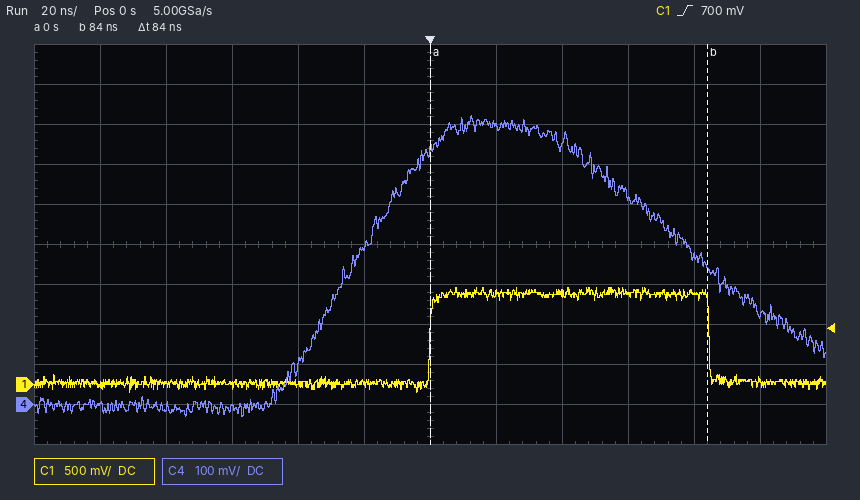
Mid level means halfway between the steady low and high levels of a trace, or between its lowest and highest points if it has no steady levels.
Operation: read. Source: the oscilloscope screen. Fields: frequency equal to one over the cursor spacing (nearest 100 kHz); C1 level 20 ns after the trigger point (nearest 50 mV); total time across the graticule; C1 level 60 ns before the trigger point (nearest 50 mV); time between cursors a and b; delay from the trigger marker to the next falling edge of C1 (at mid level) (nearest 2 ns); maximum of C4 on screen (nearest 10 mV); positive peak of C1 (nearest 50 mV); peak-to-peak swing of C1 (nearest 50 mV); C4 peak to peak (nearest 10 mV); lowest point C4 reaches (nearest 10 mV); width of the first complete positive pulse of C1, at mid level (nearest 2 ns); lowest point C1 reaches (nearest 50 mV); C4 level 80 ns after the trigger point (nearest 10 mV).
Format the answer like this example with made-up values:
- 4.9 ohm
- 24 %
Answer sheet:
- 11.9 MHz
- 1.15 V
- 240 ns
- 0 mV
- 84 ns
- 84 ns
- 720 mV
- 1.20 V
- 1.30 V
- 750 mV
- -30 mV
- 84 ns
- -100 mV
- 370 mV
